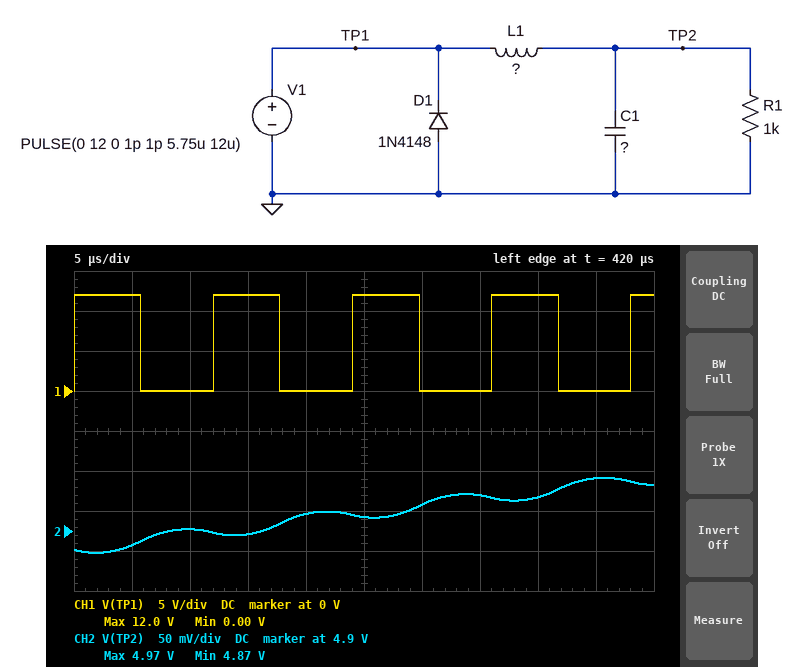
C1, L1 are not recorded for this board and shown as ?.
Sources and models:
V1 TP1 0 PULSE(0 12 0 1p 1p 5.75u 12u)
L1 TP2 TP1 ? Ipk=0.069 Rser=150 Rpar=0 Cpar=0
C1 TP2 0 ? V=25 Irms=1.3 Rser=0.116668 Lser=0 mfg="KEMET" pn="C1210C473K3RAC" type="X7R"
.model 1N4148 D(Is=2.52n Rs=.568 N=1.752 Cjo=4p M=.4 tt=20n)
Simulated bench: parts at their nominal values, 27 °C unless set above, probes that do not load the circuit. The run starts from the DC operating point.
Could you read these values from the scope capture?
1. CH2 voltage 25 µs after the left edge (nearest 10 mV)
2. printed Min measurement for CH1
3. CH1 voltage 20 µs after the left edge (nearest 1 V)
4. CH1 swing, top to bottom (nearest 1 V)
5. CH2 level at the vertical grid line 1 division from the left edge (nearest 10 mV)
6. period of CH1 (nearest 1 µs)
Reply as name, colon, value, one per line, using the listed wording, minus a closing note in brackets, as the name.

CH2 voltage 25 µs after the left edge: 4.92 V
printed Min measurement for CH1: 0.00 V
CH1 voltage 20 µs after the left edge: 0 V
CH1 swing, top to bottom: 12 V
CH2 level at the vertical grid line 1 division from the left edge: 4.88 V
period of CH1: 12 µs
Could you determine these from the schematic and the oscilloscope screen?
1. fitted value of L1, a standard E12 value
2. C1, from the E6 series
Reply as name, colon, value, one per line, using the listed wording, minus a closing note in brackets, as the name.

fitted value of L1, a standard E12 value: 47 mH
C1, from the E6 series: 68 nF
